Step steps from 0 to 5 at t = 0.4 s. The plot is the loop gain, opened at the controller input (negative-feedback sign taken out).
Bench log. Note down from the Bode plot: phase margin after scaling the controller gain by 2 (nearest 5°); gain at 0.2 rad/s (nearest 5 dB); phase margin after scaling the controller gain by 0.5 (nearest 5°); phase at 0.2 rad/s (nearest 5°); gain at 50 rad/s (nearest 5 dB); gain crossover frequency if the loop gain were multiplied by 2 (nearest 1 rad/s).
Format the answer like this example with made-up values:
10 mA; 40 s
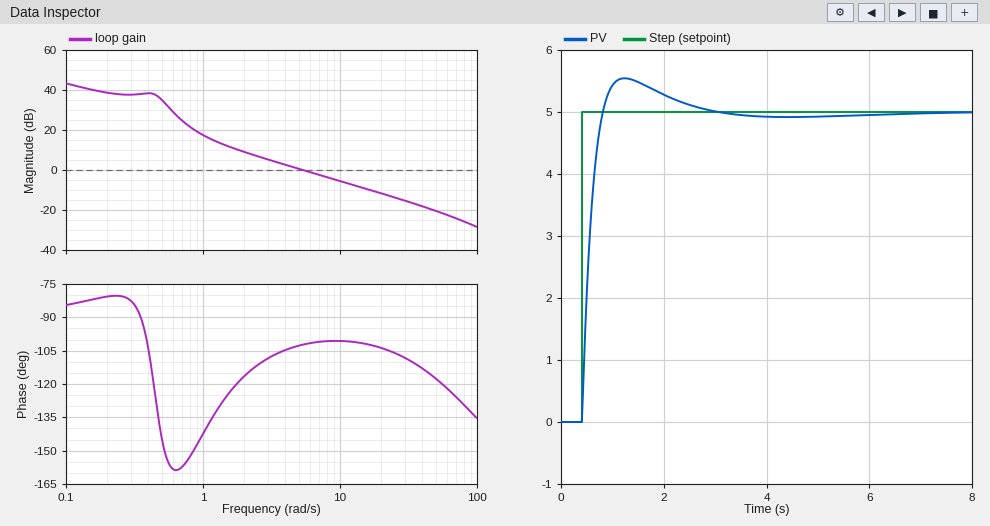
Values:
80°; 40 dB; 70°; -80°; -20 dB; 11 rad/s
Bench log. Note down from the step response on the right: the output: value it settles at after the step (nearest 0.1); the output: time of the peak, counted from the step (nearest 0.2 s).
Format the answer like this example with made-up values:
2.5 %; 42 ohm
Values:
5.0; 0.8 s
